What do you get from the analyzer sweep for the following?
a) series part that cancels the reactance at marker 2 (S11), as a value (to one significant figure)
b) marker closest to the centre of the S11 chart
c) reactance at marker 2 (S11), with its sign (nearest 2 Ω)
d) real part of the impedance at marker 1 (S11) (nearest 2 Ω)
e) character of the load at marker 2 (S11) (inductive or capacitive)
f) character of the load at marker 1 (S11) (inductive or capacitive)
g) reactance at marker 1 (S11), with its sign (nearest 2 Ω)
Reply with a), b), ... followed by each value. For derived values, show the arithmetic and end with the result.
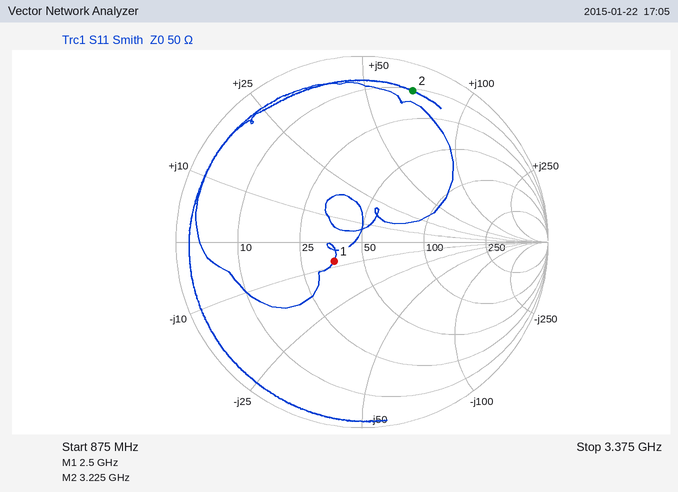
a) C = 1/(2π × 3.225 GHz × 68 Ω) ≈ 726 fF, so 700 fF to one significant figure
b) marker 1
c) +68 Ω
d) 36 Ω
e) inductive
f) capacitive
g) -8 Ω
